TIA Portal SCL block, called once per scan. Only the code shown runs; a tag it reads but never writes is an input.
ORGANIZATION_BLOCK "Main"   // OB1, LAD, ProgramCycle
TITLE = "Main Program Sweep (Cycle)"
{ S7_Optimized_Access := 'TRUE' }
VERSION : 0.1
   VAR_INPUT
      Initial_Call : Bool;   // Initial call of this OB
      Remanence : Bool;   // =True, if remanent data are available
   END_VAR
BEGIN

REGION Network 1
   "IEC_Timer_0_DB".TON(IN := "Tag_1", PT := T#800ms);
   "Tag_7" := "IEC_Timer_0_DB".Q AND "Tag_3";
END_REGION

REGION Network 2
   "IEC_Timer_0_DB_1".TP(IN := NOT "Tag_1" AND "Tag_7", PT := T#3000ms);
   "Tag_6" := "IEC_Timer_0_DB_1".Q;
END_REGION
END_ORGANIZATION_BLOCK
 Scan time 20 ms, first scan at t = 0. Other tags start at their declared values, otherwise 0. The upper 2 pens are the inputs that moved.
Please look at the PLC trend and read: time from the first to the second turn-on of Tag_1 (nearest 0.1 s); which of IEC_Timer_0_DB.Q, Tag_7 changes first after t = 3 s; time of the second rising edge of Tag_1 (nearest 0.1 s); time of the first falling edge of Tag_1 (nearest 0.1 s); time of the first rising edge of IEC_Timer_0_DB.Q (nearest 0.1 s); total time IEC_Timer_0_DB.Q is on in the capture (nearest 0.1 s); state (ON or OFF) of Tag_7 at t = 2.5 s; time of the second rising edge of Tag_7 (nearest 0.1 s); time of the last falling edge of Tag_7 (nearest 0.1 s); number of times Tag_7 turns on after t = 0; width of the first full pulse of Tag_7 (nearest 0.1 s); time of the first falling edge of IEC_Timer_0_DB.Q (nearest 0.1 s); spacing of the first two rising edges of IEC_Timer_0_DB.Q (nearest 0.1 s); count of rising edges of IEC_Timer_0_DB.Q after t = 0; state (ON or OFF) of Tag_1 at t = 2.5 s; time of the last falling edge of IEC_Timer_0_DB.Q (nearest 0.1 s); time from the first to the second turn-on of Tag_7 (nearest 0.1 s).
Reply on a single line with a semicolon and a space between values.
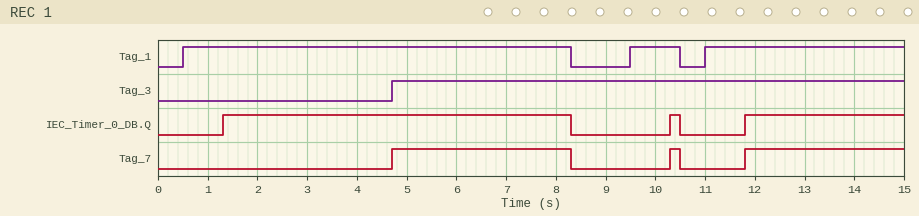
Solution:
9.0 s; Tag_7; 9.5 s; 8.3 s; 1.3 s; 10.4 s; OFF; 10.3 s; 10.5 s; 3; 3.6 s; 8.3 s; 9.0 s; 3; ON; 10.5 s; 5.6 s
